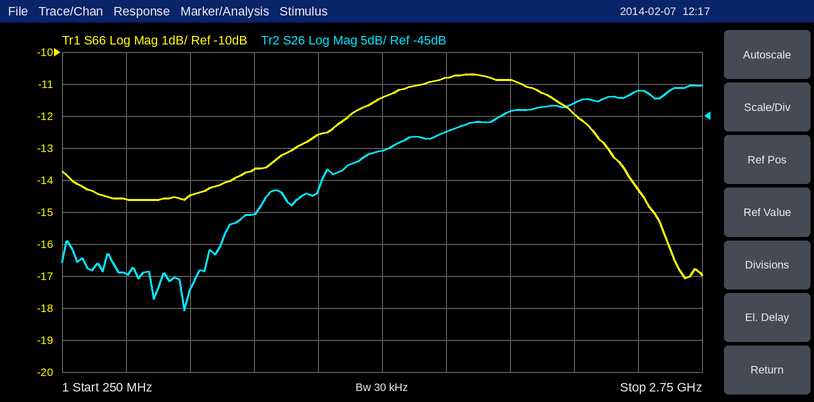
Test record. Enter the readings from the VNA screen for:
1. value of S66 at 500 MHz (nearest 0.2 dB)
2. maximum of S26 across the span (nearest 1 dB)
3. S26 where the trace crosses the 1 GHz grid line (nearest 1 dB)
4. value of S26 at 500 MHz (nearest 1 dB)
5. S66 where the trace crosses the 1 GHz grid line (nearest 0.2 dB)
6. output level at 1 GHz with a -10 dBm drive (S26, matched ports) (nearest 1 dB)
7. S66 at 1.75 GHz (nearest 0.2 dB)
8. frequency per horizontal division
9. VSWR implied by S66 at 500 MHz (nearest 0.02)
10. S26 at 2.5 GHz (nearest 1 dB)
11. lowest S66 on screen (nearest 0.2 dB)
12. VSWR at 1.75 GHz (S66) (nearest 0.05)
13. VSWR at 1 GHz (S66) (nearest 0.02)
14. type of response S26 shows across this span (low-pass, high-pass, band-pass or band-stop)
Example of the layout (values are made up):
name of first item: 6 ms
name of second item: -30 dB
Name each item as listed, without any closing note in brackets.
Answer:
value of S66 at 500 MHz: -14.6 dB
maximum of S26 across the span: -40 dB
S26 where the trace crosses the 1 GHz grid line: -60 dB
value of S26 at 500 MHz: -70 dB
S66 where the trace crosses the 1 GHz grid line: -13.6 dB
output level at 1 GHz with a -10 dBm drive (S26, matched ports): -70 dBm
S66 at 1.75 GHz: -10.8 dB
frequency per horizontal division: 250 MHz
VSWR implied by S66 at 500 MHz: 1.46
S26 at 2.5 GHz: -41 dB
lowest S66 on screen: -17.0 dB
VSWR at 1.75 GHz (S66): 1.80
VSWR at 1 GHz (S66): 1.52
type of response S26 shows across this span: high-pass
